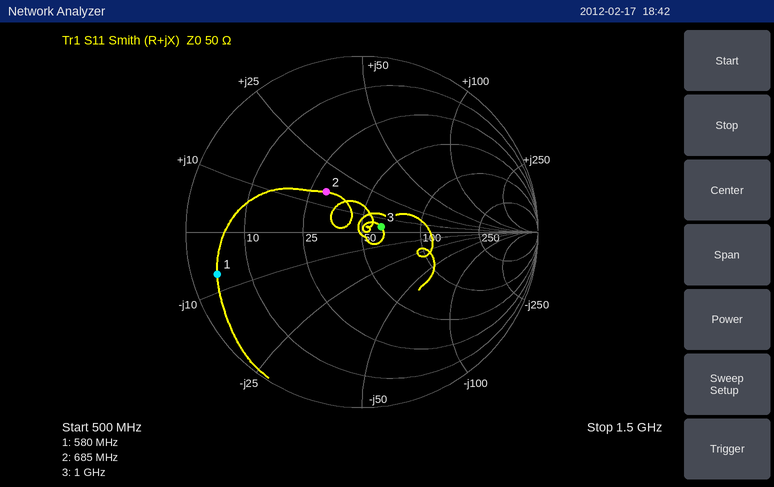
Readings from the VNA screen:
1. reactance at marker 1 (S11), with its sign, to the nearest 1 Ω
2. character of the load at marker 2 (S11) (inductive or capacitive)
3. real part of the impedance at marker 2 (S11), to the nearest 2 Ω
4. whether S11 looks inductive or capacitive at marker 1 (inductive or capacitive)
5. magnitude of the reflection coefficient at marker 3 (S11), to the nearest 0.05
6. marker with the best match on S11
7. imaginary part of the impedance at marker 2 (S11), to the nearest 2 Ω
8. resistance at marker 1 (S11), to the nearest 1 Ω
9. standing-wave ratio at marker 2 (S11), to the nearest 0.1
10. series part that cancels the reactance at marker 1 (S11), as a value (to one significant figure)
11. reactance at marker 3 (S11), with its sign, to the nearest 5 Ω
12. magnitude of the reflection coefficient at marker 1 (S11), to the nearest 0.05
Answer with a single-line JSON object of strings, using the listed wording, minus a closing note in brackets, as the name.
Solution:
{"reactance at marker 1 (S11), with its sign, to the nearest 1 Ω": "-7 Ω", "character of the load at marker 2 (S11)": "inductive", "real part of the impedance at marker 2 (S11), to the nearest 2 Ω": "30 Ω", "whether S11 looks inductive or capacitive at marker 1": "capacitive", "magnitude of the reflection coefficient at marker 3 (S11), to the nearest 0.05": "0.10", "marker with the best match on S11": "marker 3", "imaginary part of the impedance at marker 2 (S11), to the nearest 2 Ω": "+16 Ω", "resistance at marker 1 (S11), to the nearest 1 Ω": "4 Ω", "standing-wave ratio at marker 2 (S11), to the nearest 0.1": "1.9", "series part that cancels the reactance at marker 1 (S11), as a value": "2 nH", "reactance at marker 3 (S11), with its sign, to the nearest 5 Ω": "+5 Ω", "magnitude of the reflection coefficient at marker 1 (S11), to the nearest 0.05": "0.85"}
